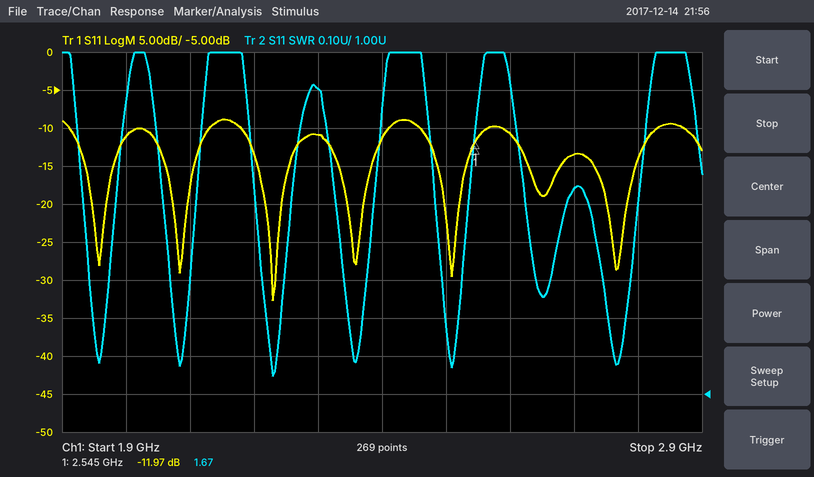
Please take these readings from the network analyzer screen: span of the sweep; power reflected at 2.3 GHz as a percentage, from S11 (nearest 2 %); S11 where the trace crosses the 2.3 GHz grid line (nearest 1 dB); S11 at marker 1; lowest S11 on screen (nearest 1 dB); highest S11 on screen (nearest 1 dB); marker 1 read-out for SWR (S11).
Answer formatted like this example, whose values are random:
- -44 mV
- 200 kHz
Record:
- 1 GHz
- 8 %
- -11 dB
- -11.97 dB
- -33 dB
- -9 dB
- 1.67
